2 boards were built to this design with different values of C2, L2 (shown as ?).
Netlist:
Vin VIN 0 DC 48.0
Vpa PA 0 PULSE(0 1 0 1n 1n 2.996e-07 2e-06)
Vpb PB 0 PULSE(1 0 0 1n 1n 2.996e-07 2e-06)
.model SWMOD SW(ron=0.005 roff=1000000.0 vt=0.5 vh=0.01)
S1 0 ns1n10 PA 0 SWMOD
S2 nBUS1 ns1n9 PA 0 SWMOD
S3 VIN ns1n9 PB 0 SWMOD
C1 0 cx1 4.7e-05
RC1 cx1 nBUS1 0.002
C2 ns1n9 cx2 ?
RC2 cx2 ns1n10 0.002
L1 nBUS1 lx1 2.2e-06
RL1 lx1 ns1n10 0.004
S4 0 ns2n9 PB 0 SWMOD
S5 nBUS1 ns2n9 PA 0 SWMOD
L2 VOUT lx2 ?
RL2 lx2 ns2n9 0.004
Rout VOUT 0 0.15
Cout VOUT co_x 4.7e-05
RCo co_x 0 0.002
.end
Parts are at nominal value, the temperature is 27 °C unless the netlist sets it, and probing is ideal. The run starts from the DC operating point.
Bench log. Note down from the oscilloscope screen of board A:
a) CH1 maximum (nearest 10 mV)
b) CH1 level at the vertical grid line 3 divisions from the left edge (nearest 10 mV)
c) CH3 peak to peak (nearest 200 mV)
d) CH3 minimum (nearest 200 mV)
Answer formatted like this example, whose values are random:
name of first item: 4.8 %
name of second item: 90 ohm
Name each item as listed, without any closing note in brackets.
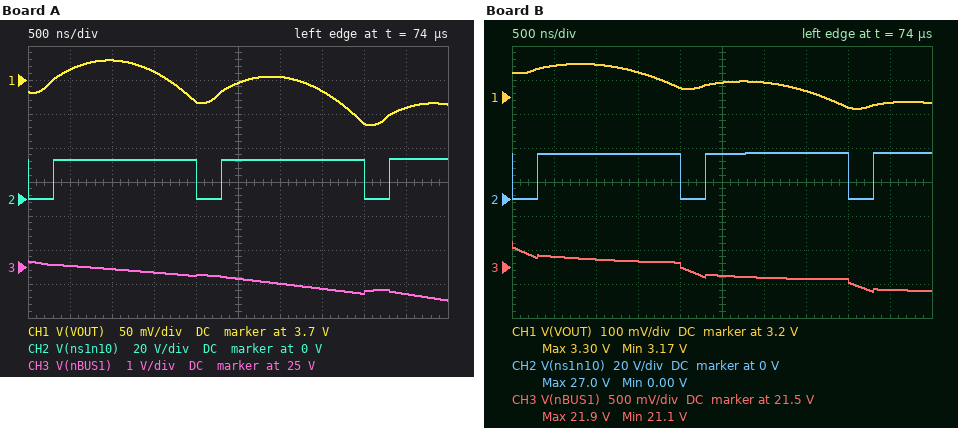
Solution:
CH1 maximum: 3.73 V
CH1 level at the vertical grid line 3 divisions from the left edge: 3.71 V
CH3 peak to peak: 1.2 V
CH3 minimum: 24.0 V
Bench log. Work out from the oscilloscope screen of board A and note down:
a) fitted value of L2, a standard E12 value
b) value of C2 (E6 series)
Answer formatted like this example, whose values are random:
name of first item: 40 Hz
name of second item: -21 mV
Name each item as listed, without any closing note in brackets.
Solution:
fitted value of L2, a standard E12 value: 680 nH
value of C2: 150 µF
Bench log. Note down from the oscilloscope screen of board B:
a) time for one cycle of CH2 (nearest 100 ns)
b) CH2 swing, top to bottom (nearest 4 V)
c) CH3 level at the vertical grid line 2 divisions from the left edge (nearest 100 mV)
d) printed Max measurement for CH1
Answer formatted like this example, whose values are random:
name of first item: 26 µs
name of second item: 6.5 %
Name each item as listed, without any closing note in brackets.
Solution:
time for one cycle of CH2: 2.0 µs
CH2 swing, top to bottom: 28 V
CH3 level at the vertical grid line 2 divisions from the left edge: 21.6 V
printed Max measurement for CH1: 3.30 V
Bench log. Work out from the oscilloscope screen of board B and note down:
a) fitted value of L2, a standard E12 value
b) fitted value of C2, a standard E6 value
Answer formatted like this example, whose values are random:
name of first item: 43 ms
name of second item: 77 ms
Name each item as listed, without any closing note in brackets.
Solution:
fitted value of L2, a standard E12 value: 680 nH
fitted value of C2, a standard E6 value: 15 µF
